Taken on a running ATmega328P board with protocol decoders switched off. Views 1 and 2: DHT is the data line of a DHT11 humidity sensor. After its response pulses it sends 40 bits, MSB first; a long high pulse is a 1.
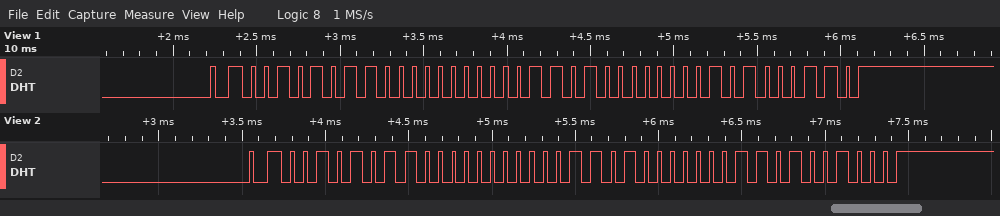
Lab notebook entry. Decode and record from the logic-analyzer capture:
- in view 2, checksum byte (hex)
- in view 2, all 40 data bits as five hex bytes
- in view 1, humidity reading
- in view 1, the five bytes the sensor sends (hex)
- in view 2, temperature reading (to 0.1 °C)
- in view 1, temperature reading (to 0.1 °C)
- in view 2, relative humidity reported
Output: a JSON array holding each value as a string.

["0x48", "2B 00 1A 03 48", "43 %", "2B 00 1A 01 46", "26.3 °C", "26.1 °C", "43 %"]
